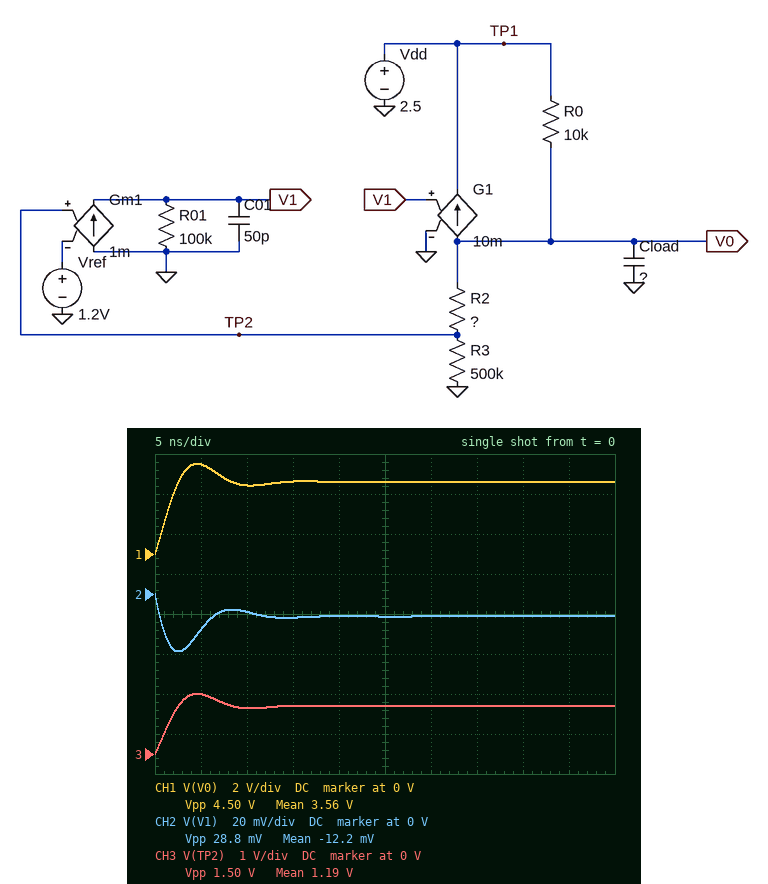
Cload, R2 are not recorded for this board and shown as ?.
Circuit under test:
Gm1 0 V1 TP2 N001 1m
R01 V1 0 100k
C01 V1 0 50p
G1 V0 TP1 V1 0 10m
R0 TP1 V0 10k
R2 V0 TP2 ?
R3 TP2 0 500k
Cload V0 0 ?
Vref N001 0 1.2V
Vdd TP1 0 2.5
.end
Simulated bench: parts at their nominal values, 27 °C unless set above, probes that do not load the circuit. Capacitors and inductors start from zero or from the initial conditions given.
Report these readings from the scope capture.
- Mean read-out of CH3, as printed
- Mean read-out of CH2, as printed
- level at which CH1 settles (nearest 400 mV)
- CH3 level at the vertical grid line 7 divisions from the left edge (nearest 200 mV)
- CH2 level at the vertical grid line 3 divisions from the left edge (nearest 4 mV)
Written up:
1.19 V
-12.2 mV
3.6 V
1.2 V
-12 mV
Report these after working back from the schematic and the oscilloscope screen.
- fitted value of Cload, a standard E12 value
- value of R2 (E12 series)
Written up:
180 fF
1 MΩ
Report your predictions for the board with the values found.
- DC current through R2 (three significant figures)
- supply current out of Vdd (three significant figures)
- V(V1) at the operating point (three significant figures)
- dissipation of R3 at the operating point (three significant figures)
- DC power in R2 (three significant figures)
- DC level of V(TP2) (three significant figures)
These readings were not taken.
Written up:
2.40 µA
2.40 µA
-11.2 mV
2.88 µW
5.76 µW
1.20 V
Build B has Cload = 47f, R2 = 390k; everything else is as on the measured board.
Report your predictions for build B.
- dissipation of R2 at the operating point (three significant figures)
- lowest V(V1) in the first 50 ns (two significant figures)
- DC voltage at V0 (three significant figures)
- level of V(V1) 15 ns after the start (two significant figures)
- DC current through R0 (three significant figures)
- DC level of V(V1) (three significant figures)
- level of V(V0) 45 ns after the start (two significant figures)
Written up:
2.25 µW
-6.1 mV
2.14 V
3.4 mV
36.4 µA
3.40 mV
2.1 V
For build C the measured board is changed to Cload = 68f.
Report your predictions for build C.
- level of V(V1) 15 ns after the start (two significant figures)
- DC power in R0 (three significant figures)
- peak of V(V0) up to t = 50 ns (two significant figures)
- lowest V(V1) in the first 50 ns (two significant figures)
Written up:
-11 mV
121 µW
3.9 V
-16 mV
